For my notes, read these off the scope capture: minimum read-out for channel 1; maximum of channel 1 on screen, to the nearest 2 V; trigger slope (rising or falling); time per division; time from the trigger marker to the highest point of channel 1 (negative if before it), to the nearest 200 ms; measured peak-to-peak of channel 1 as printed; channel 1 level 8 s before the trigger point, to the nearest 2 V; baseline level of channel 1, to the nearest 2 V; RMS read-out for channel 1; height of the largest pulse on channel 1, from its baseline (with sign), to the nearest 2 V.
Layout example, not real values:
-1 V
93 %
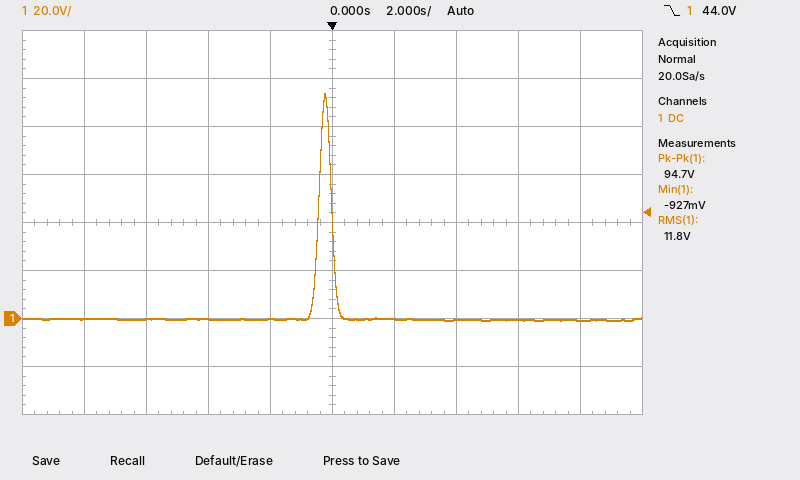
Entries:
-927 mV
94 V
falling
2 s
-200 ms
94.7 V
0 V
0 V
11.8 V
+94 V
